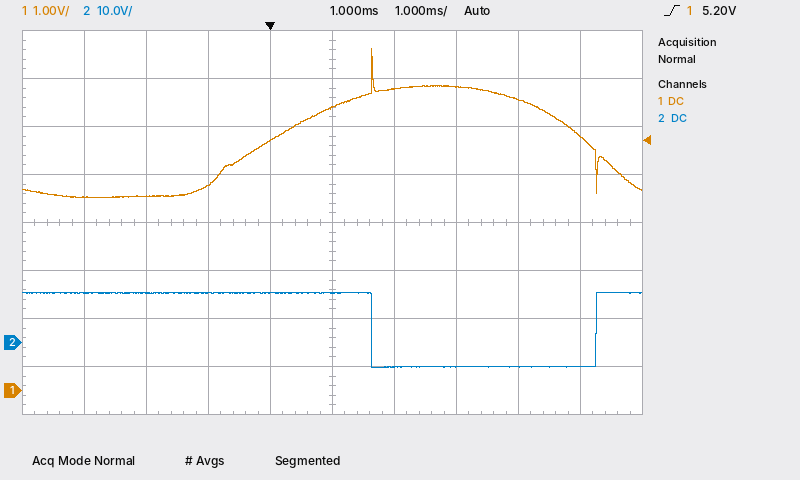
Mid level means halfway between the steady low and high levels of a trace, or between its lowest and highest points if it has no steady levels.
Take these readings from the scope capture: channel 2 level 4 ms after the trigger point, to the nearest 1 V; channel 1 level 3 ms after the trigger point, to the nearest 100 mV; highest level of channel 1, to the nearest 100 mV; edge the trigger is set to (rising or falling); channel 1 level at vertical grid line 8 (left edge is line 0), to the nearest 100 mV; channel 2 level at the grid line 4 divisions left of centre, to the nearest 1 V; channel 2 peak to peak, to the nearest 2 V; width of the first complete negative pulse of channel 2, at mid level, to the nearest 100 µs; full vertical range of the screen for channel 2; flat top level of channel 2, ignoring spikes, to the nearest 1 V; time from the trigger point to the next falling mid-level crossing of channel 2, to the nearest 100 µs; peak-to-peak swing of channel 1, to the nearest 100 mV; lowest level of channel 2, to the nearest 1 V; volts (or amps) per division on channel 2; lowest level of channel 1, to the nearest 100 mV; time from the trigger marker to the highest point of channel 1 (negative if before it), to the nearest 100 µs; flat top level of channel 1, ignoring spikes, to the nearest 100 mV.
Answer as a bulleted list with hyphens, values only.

- -5 V
- 6.3 V
- 7.1 V
- rising
- 6.1 V
- 10 V
- 16 V
- 3.6 ms
- 80 V
- 10 V
- 1.6 ms
- 3.1 V
- -5 V
- 10 V
- 4.0 V
- +1.6 ms
- 6.3 V
